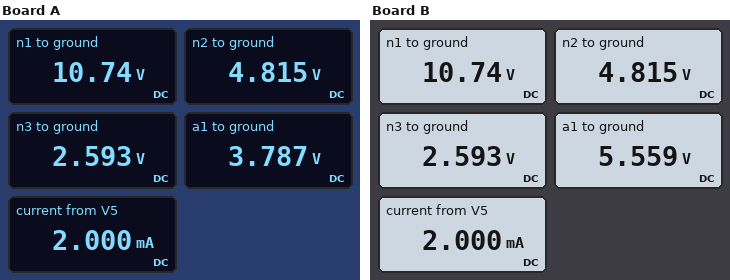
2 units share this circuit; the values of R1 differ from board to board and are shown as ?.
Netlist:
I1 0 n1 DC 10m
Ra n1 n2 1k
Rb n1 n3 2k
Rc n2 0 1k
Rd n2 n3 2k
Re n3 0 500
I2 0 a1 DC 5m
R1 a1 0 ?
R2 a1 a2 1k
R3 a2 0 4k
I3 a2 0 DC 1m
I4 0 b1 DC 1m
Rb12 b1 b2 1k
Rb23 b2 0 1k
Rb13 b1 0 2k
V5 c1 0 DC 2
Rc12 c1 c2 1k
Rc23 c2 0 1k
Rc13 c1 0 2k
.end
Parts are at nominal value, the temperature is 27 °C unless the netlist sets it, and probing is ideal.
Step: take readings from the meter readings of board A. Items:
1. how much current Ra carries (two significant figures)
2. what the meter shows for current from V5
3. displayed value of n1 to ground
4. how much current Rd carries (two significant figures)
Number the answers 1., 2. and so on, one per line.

1. 5.9 mA
2. 2.000 mA
3. 10.74 V
4. 1.1 mA
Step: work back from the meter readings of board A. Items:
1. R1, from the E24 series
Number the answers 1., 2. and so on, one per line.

1. 1.1 kΩ
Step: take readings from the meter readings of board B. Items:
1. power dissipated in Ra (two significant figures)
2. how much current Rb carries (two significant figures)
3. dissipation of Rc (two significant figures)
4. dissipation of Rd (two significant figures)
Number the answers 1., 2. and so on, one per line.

1. 35 mW
2. 4.1 mA
3. 23 mW
4. 2.5 mW
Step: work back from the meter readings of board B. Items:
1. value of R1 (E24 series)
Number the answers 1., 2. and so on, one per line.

1. 1.8 kΩ
